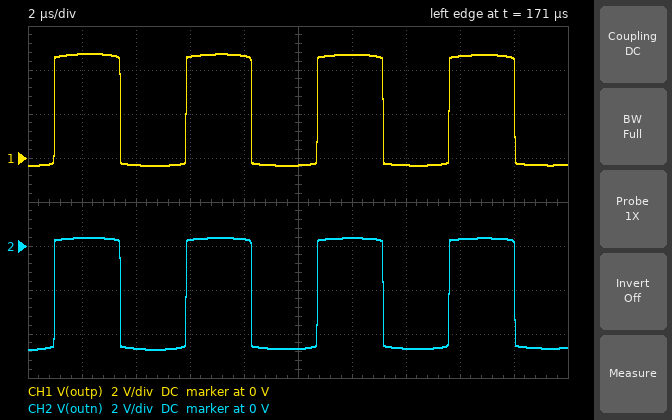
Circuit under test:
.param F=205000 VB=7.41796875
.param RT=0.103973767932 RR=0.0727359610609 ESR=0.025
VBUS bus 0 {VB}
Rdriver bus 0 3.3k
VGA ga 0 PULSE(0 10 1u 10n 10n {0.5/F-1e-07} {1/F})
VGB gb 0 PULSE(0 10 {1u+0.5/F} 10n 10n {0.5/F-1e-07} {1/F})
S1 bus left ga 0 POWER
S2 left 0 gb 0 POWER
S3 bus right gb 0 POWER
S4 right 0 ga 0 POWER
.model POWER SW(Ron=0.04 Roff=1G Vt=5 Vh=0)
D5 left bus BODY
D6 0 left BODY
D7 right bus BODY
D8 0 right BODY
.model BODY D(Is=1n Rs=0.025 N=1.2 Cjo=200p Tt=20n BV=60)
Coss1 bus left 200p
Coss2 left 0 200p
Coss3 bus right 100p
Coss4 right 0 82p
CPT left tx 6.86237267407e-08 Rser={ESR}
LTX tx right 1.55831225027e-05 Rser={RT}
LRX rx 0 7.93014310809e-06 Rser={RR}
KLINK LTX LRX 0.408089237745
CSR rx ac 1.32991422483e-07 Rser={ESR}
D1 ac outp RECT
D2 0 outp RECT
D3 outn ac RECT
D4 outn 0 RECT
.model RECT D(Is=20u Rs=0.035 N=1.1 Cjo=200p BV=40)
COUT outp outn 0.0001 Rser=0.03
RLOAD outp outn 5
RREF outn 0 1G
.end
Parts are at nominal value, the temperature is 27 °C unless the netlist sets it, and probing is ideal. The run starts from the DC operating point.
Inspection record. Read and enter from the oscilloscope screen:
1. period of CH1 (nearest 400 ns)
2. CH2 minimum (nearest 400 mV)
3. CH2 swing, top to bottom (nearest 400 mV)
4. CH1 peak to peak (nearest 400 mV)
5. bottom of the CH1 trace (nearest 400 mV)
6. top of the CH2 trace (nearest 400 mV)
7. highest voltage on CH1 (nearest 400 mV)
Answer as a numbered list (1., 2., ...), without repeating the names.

1. 4.8 µs
2. -4.8 V
3. 5.2 V
4. 5.2 V
5. -400 mV
6. 400 mV
7. 4.8 V
